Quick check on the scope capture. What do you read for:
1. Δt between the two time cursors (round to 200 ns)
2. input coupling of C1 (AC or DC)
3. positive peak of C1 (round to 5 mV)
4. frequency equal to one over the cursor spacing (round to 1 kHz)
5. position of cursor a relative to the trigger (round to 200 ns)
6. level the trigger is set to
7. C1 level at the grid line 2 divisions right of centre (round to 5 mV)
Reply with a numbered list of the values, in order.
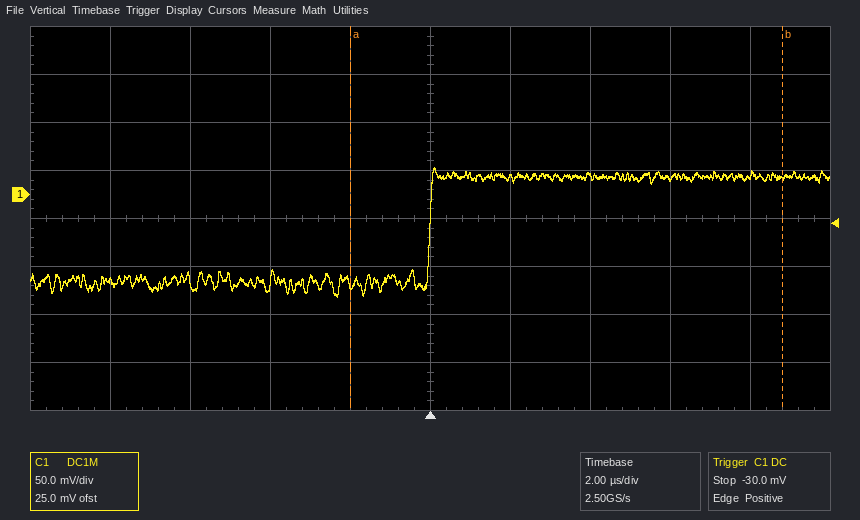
1. 10.8 µs
2. DC
3. 30 mV
4. 93 kHz
5. -2.0 µs
6. -30.0 mV
7. 20 mV
